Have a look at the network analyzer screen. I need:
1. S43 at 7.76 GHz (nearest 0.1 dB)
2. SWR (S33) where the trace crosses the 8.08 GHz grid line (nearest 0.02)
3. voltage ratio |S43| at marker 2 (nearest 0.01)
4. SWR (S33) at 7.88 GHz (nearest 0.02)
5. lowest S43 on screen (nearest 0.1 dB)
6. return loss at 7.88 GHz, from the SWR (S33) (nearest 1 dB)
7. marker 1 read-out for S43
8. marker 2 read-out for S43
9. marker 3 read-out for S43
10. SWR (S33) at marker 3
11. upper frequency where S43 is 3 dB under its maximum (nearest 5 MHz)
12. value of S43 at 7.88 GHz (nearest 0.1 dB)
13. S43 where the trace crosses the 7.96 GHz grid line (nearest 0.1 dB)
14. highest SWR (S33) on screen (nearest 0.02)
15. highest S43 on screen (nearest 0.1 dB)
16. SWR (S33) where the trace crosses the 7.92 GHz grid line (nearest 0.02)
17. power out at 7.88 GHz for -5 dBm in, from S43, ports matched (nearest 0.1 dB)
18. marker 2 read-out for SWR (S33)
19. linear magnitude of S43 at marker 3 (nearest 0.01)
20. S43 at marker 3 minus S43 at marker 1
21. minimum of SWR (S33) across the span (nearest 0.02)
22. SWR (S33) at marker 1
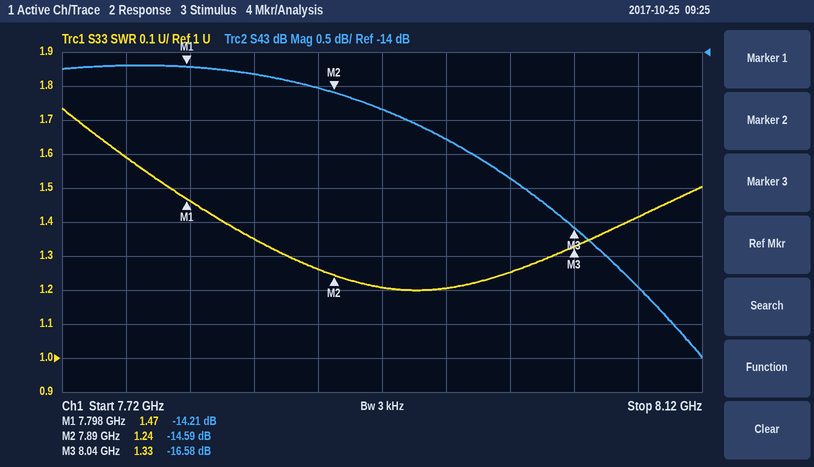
-14.2 dB
1.42
0.19
1.26
-18.5 dB
19 dB
-14.21 dB
-14.59 dB
-16.58 dB
1.33
8.070 GHz
-14.5 dB
-15.3 dB
1.74
-14.2 dB
1.20
-19.5 dBm
1.24
0.15
-2.37 dB
1.20
1.47
